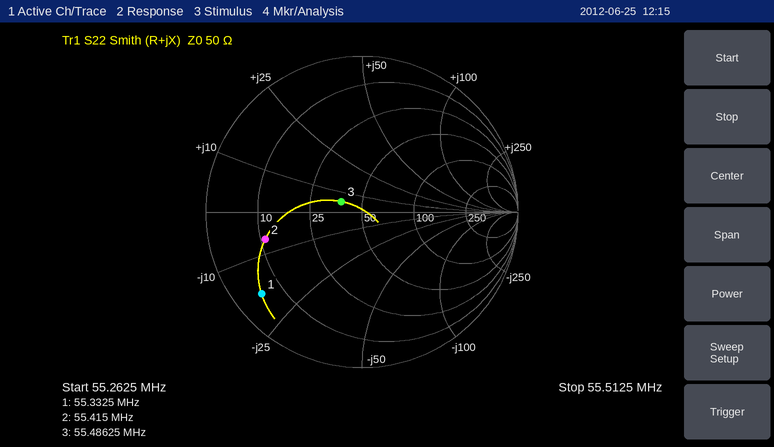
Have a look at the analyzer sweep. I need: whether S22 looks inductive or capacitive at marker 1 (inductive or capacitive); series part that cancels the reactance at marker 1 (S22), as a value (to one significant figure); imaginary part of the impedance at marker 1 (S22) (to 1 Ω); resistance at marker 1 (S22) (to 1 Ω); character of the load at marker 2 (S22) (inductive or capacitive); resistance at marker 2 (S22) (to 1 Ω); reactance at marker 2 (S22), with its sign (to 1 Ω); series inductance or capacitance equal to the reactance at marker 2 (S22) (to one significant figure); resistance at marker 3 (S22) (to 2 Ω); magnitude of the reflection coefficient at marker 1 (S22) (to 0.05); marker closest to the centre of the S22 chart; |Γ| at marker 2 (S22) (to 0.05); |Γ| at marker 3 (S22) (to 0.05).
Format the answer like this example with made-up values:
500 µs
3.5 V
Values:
capacitive
50 nH
-18 Ω
5 Ω
capacitive
11 Ω
-7 Ω
400 pF
38 Ω
0.85
marker 3
0.65
0.15
